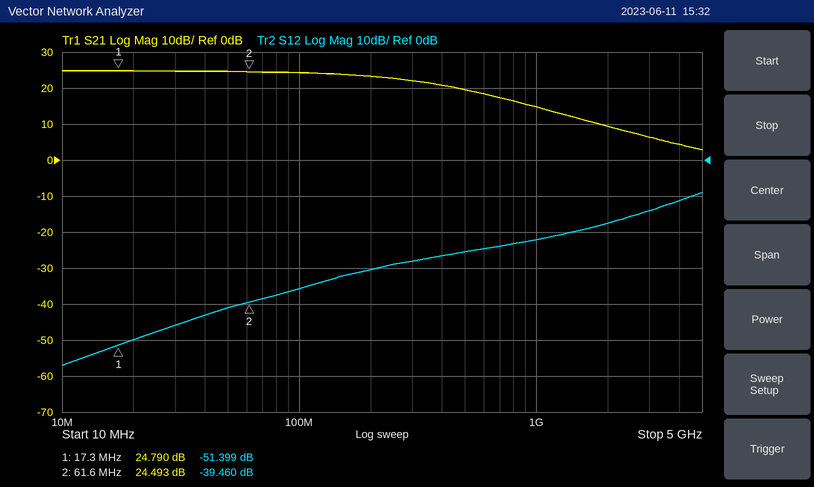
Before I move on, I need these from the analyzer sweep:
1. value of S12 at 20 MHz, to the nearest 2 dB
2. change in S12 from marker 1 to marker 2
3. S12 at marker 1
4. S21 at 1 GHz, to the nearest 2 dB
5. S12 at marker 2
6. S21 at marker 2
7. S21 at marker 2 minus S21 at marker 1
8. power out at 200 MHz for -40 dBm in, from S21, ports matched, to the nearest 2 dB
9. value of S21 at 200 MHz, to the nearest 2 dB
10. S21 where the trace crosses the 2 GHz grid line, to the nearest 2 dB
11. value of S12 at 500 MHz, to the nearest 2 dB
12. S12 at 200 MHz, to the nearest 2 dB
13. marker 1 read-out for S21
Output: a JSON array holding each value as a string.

["-50 dB", "11.939 dB", "-51.399 dB", "14 dB", "-39.460 dB", "24.493 dB", "-0.297 dB", "-16 dBm", "24 dB", "10 dB", "-26 dB", "-30 dB", "24.790 dB"]
